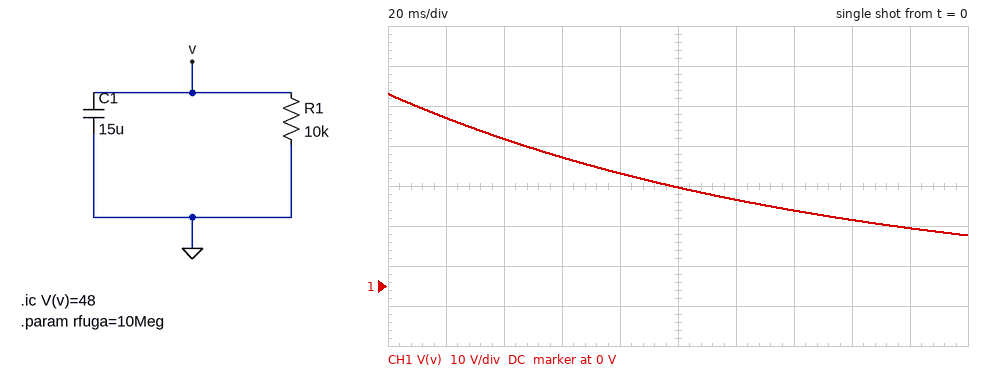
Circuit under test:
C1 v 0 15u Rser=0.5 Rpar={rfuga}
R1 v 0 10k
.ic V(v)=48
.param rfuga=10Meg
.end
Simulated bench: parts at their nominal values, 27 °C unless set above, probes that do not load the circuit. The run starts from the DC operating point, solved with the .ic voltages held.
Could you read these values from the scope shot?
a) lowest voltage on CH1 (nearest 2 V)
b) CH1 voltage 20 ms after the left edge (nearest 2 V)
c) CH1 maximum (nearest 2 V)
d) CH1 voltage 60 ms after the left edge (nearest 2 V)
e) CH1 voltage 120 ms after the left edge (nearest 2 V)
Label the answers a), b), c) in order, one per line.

a) 12 V
b) 42 V
c) 48 V
d) 32 V
e) 22 V
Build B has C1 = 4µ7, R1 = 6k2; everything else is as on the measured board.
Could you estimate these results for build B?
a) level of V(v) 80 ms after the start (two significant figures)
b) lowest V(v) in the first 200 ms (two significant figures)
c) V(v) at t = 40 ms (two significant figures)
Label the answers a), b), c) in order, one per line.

a) 3.1 V
b) 50 mV
c) 12 V
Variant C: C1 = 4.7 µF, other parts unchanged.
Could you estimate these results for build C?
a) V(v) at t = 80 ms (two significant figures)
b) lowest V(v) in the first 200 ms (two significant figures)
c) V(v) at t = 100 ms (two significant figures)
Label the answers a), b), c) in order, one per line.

a) 8.7 V
b) 680 mV
c) 5.7 V
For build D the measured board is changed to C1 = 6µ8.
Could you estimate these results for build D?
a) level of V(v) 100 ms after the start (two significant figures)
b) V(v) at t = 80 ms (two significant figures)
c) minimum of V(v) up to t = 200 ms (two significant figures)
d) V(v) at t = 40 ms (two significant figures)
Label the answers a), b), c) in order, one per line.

a) 11 V
b) 15 V
c) 2.5 V
d) 27 V
